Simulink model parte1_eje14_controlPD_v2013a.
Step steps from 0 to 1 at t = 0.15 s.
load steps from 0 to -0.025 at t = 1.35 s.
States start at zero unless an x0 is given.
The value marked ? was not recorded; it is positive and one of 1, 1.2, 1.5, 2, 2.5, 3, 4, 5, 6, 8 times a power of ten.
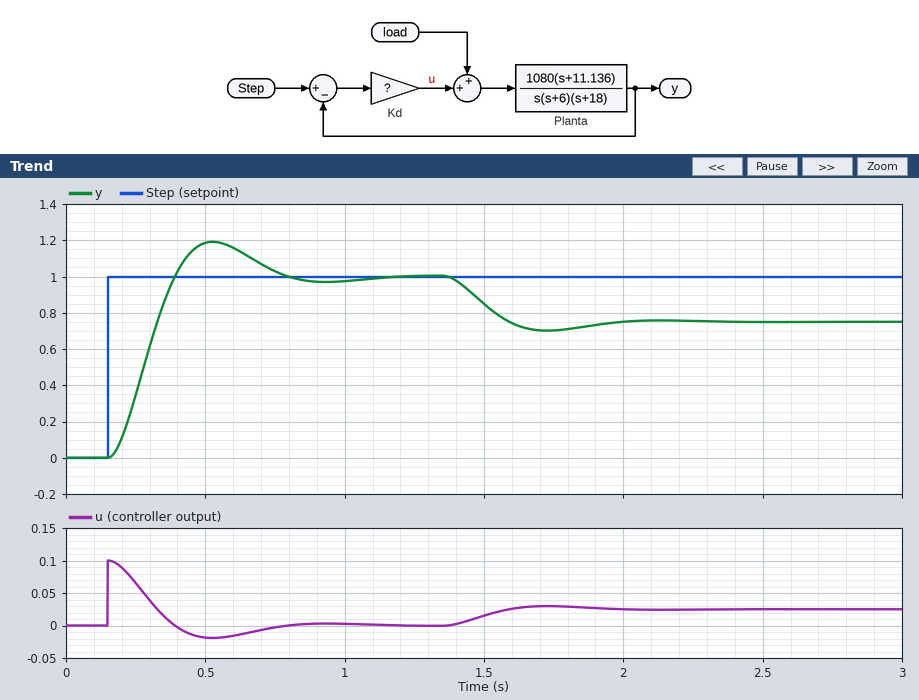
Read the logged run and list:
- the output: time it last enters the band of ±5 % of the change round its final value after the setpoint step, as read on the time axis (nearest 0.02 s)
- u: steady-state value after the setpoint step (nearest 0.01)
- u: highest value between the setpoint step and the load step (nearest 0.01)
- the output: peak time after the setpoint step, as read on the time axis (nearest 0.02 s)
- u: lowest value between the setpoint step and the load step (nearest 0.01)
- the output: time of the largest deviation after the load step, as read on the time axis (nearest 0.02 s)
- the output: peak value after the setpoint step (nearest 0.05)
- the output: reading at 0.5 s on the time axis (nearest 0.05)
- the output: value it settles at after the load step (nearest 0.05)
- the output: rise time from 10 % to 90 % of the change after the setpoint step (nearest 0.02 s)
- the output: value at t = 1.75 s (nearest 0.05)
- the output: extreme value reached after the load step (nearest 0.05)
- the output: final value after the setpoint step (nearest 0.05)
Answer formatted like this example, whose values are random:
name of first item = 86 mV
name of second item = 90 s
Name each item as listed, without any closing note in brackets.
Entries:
the output: time it last enters the band of ±5 % of the change round its final value after the setpoint step, as read on the time axis = 0.72 s
u: steady-state value after the setpoint step = 0.00
u: highest value between the setpoint step and the load step = 0.10
the output: peak time after the setpoint step, as read on the time axis = 0.52 s
u: lowest value between the setpoint step and the load step = -0.02
the output: time of the largest deviation after the load step, as read on the time axis = 1.72 s
the output: peak value after the setpoint step = 1.20
the output: reading at 0.5 s on the time axis = 1.20
the output: value it settles at after the load step = 0.75
the output: rise time from 10 % to 90 % of the change after the setpoint step = 0.16 s
the output: value at t = 1.75 s = 0.70
the output: extreme value reached after the load step = 0.70
the output: final value after the setpoint step = 1.00
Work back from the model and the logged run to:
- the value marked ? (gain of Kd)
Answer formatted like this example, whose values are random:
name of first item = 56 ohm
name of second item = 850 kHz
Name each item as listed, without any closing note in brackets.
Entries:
the value marked ? = 0.1
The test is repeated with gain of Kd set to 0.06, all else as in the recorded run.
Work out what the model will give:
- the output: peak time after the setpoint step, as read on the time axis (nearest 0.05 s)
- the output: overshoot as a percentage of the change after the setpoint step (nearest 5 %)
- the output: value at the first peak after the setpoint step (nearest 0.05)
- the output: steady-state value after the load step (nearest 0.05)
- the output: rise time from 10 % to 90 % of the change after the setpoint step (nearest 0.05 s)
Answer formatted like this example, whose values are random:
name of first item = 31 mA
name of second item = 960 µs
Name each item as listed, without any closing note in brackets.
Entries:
the output: peak time after the setpoint step, as read on the time axis = 0.70 s
the output: overshoot as a percentage of the change after the setpoint step = 10 %
the output: value at the first peak after the setpoint step = 1.10
the output: steady-state value after the load step = 0.60
the output: rise time from 10 % to 90 % of the change after the setpoint step = 0.25 s
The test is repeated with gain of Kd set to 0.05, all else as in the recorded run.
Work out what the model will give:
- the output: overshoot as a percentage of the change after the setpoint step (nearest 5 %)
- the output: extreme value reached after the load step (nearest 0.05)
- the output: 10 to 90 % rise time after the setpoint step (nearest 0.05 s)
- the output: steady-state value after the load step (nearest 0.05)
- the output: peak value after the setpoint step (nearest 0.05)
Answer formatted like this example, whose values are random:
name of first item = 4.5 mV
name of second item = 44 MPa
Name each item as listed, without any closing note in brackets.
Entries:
the output: overshoot as a percentage of the change after the setpoint step = 10 %
the output: extreme value reached after the load step = 0.45
the output: 10 to 90 % rise time after the setpoint step = 0.30 s
the output: steady-state value after the load step = 0.50
the output: peak value after the setpoint step = 1.10
